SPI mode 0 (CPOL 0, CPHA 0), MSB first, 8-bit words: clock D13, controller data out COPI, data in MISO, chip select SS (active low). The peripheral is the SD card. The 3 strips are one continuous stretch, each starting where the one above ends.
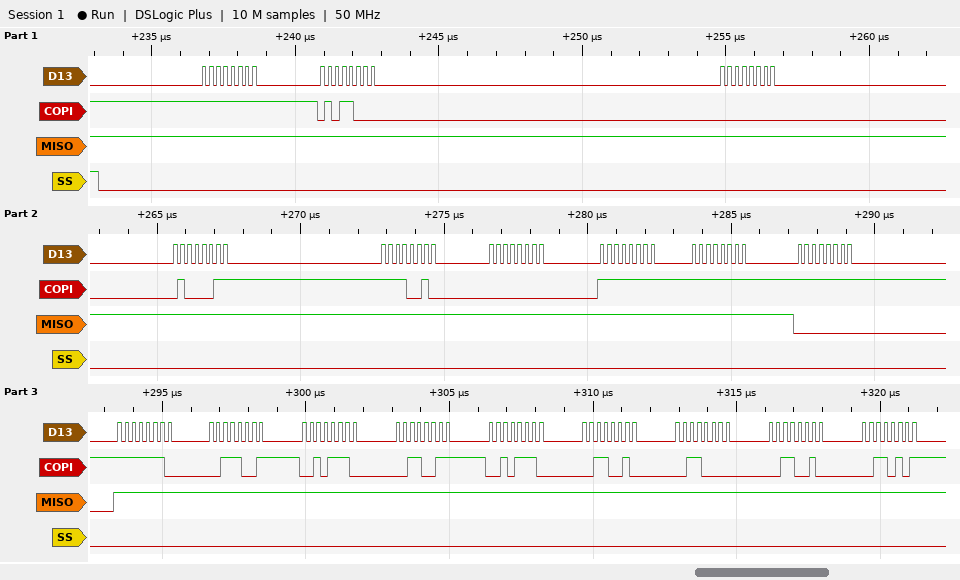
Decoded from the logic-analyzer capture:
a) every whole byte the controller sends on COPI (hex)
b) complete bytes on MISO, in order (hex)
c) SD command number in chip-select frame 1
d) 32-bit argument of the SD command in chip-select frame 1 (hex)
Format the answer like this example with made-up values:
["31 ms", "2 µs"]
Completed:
["FF 58 00 43 F2 00 FF FF FF FE 39 2E 33 2E 32 30 32 35", "FF FF FF FF FF FF FF FF 00 FF FF FF FF FF FF FF FF FF", "CMD24", "0x0043F200"]
